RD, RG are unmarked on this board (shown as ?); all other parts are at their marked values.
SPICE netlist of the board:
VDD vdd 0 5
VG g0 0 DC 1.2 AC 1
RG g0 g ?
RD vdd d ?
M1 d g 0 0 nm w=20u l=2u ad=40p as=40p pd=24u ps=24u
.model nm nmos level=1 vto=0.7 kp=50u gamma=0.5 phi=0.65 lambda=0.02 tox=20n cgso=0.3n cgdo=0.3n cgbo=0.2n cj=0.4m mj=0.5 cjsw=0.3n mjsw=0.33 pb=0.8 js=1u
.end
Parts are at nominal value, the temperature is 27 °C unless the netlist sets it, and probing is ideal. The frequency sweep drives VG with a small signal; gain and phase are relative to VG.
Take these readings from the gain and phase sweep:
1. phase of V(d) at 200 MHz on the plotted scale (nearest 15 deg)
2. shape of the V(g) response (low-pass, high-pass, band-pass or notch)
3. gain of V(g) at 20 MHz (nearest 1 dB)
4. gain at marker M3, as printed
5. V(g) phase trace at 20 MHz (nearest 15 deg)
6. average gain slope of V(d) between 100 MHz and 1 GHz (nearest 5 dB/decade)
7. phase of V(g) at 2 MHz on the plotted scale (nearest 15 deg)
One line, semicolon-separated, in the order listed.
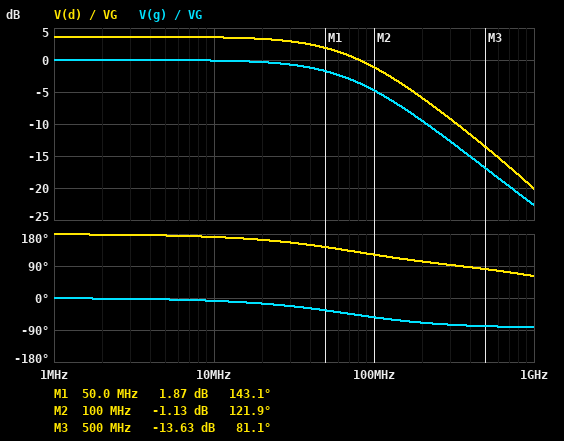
105 deg; low-pass; 0 dB; -13.63 dB; -15 deg; -20 dB/decade; 0 deg
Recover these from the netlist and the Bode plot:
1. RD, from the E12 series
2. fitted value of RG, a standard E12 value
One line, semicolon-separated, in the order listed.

5.6 kΩ; 33 kΩ
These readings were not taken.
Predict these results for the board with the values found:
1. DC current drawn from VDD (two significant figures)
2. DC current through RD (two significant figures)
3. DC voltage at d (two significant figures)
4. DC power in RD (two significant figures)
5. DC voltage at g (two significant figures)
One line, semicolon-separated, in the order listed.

68 µA; 68 µA; 4.6 V; 26 µW; 1.2 V
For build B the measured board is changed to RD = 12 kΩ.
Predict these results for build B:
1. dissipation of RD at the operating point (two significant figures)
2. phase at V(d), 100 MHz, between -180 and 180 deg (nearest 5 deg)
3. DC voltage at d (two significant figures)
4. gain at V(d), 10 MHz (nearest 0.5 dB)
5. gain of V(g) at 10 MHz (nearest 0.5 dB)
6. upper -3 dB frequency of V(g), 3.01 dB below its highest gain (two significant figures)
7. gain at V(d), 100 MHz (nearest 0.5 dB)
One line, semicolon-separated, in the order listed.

55 µW; 115 deg; 4.2 V; 10.0 dB; 0 dB; 61 MHz; 4.5 dB
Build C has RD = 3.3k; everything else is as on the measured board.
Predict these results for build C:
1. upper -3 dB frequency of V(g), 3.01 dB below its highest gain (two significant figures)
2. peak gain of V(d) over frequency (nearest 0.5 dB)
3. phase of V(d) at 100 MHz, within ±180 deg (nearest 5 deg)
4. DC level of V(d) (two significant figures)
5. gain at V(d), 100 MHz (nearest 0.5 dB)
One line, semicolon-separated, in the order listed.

75 MHz; -1.0 dB; 125 deg; 4.8 V; -5.5 dB
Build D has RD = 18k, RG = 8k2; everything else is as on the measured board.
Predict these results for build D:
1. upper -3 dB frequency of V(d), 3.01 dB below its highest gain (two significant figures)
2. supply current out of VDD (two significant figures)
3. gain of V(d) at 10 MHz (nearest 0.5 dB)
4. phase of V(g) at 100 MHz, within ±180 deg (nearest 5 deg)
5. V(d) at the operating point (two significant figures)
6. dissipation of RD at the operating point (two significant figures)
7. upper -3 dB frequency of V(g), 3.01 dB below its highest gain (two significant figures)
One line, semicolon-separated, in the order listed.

180 MHz; 67 µA; 13.5 dB; -25 deg; 3.8 V; 81 µW; 210 MHz
